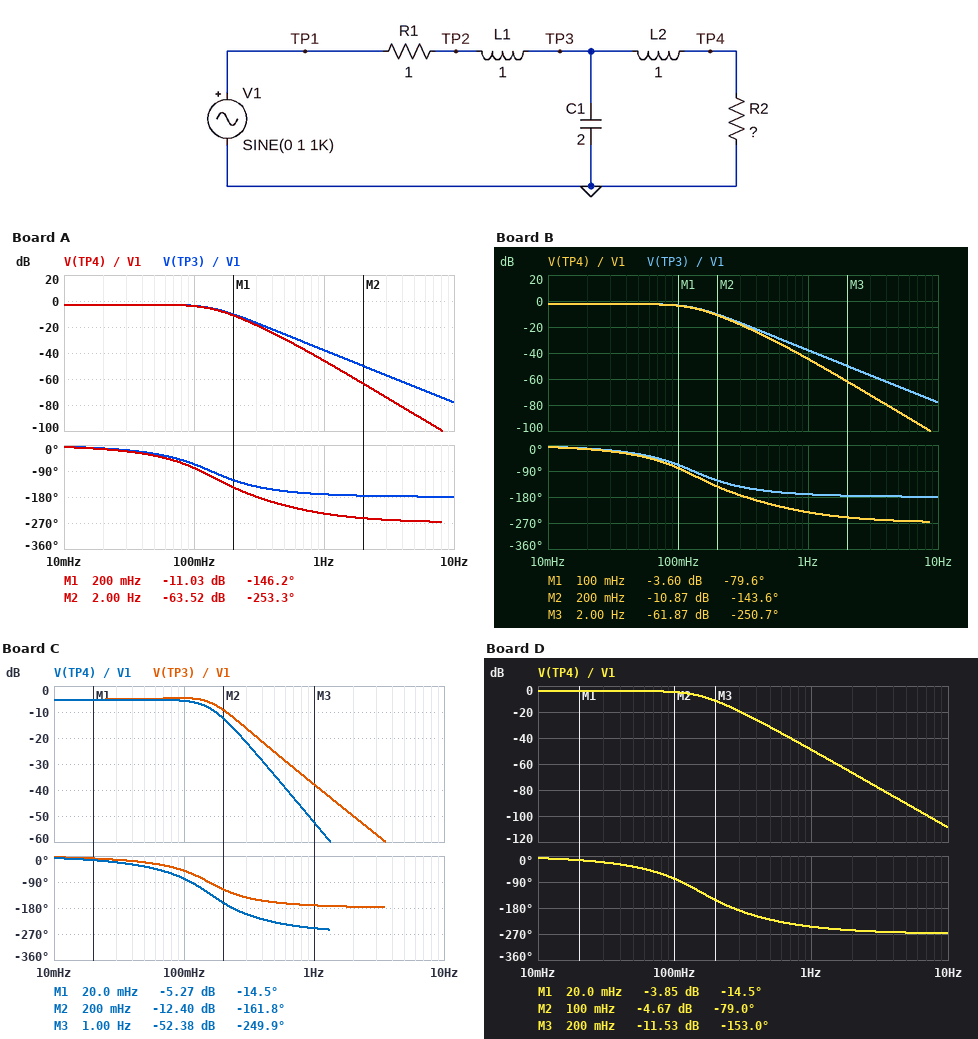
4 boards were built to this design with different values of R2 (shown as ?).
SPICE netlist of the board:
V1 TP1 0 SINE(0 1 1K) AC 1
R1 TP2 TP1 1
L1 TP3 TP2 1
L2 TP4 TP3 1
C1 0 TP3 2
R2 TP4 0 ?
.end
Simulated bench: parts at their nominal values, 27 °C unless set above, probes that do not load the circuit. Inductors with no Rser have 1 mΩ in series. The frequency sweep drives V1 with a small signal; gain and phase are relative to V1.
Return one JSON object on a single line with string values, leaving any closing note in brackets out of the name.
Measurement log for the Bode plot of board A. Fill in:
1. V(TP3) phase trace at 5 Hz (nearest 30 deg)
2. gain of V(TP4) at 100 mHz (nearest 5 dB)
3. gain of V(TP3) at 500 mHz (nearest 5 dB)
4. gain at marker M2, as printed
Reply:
{"V(TP3) phase trace at 5 Hz": "-180 deg", "gain of V(TP4) at 100 mHz": "-5 dB", "gain of V(TP3) at 500 mHz": "-25 dB", "gain at marker M2, as printed": "-63.52 dB"}
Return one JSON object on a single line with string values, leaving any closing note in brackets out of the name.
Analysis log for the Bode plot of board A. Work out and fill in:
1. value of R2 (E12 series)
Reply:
{"value of R2": "2.7 Ω"}
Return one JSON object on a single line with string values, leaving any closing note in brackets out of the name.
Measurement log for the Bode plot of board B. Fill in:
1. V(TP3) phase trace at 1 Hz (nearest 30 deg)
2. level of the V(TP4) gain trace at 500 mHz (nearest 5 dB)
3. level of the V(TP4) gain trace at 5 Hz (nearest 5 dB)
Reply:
{"V(TP3) phase trace at 1 Hz": "-180 deg", "level of the V(TP4) gain trace at 500 mHz": "-30 dB", "level of the V(TP4) gain trace at 5 Hz": "-85 dB"}
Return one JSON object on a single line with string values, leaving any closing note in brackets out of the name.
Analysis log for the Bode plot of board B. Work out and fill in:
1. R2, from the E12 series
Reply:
{"R2, from the E12 series": "3.3 Ω"}
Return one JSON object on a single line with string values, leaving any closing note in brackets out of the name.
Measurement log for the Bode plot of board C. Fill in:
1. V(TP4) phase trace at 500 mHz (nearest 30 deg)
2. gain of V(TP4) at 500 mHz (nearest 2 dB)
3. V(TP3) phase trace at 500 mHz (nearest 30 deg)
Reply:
{"V(TP4) phase trace at 500 mHz": "-240 deg", "gain of V(TP4) at 500 mHz": "-34 dB", "V(TP3) phase trace at 500 mHz": "-150 deg"}
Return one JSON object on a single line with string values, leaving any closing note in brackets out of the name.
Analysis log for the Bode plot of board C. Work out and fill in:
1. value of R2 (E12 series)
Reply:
{"value of R2": "1.2 Ω"}
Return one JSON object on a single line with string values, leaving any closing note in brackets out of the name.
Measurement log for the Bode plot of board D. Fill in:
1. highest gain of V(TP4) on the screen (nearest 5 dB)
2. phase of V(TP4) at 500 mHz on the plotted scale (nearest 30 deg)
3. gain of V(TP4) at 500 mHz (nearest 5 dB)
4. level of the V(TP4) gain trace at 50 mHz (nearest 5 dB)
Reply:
{"highest gain of V(TP4) on the screen": "-5 dB", "phase of V(TP4) at 500 mHz on the plotted scale": "-210 deg", "gain of V(TP4) at 500 mHz": "-30 dB", "level of the V(TP4) gain trace at 50 mHz": "-5 dB"}
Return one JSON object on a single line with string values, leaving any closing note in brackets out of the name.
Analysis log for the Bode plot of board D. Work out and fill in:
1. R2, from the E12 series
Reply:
{"R2, from the E12 series": "1.8 Ω"}
